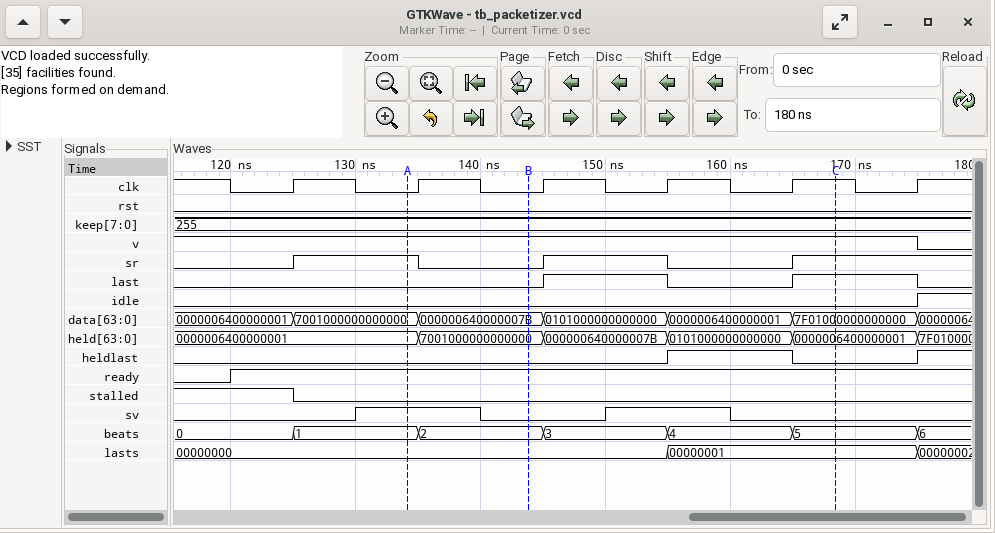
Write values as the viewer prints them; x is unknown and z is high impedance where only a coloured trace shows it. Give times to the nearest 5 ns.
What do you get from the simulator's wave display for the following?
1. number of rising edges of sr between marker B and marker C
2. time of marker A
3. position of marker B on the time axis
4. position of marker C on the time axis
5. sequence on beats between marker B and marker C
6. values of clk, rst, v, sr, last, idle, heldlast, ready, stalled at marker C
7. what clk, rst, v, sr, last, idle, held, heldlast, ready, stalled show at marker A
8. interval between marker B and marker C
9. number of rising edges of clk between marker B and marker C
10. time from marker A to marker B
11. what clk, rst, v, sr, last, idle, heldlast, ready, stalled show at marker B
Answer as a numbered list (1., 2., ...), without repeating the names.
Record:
1. 2
2. 135 ns
3. 145 ns
4. 170 ns
5. 2, 3, 4, 5
6. clk=1, rst=0, v=1, sr=1, last=1, idle=0, heldlast=0, ready=1, stalled=0
7. clk=0, rst=0, v=1, sr=1, last=0, idle=0, held=0000006400000001, heldlast=0, ready=1, stalled=0
8. 25 ns
9. 3
10. 10 ns
11. clk=0, rst=0, v=1, sr=0, last=0, idle=0, heldlast=0, ready=1, stalled=0
